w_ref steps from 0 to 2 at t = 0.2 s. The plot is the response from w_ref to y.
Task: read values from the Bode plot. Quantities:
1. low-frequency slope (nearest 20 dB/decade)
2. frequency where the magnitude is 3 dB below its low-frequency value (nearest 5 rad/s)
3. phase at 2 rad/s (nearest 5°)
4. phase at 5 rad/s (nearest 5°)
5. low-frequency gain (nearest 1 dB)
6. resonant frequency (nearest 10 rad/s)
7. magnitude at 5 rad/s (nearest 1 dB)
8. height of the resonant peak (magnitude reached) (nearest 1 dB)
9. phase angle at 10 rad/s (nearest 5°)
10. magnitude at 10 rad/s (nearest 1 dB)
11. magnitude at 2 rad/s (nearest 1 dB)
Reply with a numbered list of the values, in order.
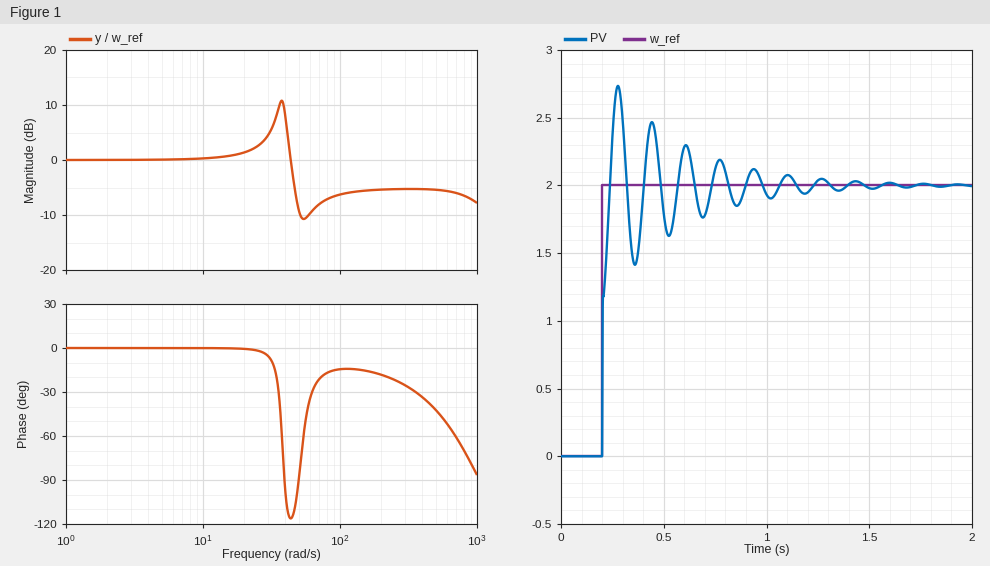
1. 0 dB/decade
2. 45 rad/s
3. 0°
4. 0°
5. 0 dB
6. 40 rad/s
7. 0 dB
8. 11 dB
9. 0°
10. 0 dB
11. 0 dB
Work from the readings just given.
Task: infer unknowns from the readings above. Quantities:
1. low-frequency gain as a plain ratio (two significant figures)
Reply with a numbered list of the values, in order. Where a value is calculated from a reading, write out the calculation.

1. 10^(0 / 20) = 1.0
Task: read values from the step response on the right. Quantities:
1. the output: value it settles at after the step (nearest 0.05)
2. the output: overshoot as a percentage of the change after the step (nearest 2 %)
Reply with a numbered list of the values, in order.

1. 2.00
2. 36 %
